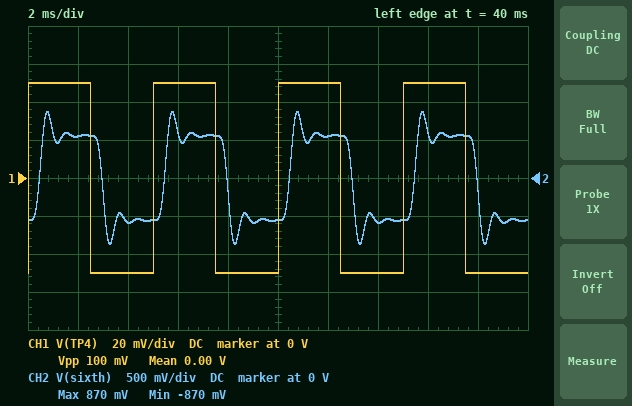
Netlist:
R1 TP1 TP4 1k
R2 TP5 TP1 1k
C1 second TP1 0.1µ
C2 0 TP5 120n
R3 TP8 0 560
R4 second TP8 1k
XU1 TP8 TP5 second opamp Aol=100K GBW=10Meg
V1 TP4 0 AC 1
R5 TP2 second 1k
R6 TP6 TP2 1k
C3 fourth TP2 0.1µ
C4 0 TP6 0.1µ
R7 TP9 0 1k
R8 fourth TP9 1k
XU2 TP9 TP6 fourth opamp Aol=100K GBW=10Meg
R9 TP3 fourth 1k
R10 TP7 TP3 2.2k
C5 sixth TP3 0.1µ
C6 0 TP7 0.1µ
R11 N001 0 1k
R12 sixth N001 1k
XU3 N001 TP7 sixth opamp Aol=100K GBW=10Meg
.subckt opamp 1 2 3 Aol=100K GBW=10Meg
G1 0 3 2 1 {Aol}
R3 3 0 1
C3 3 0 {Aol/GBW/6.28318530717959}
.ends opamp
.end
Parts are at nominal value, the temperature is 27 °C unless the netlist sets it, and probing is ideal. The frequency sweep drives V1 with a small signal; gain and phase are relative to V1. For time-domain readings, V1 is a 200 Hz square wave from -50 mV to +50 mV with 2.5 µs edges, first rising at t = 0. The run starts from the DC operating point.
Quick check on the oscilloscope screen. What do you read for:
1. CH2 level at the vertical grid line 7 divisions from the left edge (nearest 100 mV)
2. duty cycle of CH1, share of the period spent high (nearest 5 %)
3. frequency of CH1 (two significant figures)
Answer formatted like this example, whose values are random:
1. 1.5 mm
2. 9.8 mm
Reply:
1. -600 mV
2. 50 %
3. 200 Hz
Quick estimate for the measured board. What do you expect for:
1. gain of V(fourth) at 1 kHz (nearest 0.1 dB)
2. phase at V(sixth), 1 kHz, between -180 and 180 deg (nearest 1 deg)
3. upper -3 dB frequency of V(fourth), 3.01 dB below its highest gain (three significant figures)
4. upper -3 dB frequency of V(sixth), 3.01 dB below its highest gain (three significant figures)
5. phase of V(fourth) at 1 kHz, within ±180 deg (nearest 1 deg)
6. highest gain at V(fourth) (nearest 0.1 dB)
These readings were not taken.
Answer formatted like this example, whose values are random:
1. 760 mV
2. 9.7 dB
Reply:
1. 19.8 dB
2. -167 deg
3. 1.61 kHz
4. 1.45 kHz
5. -82 deg
6. 21.4 dB
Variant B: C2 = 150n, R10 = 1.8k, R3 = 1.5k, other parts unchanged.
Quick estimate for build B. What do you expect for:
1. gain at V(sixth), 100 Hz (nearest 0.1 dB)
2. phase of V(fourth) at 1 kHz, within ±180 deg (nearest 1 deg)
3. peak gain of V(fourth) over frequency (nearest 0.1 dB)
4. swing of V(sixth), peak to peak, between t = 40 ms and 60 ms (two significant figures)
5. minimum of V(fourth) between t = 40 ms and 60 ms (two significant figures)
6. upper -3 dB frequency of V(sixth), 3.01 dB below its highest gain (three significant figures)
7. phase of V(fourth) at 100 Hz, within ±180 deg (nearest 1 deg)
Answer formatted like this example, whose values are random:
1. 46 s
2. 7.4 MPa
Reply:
1. 16.5 dB
2. -121 deg
3. 10.5 dB
4. 730 mV
5. -170 mV
6. 921 Hz
7. -12 deg
